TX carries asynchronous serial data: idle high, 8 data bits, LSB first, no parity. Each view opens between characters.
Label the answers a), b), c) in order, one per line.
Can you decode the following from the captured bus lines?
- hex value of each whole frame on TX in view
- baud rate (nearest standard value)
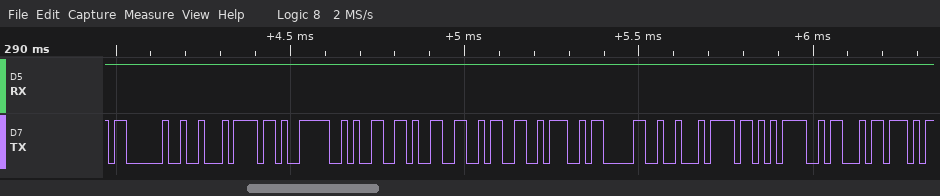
a) 03, 12, 6F, 3E, 99, 99, 9A, 3A, 83, 12, 6F, 3D, A3
b) 57600 baud
